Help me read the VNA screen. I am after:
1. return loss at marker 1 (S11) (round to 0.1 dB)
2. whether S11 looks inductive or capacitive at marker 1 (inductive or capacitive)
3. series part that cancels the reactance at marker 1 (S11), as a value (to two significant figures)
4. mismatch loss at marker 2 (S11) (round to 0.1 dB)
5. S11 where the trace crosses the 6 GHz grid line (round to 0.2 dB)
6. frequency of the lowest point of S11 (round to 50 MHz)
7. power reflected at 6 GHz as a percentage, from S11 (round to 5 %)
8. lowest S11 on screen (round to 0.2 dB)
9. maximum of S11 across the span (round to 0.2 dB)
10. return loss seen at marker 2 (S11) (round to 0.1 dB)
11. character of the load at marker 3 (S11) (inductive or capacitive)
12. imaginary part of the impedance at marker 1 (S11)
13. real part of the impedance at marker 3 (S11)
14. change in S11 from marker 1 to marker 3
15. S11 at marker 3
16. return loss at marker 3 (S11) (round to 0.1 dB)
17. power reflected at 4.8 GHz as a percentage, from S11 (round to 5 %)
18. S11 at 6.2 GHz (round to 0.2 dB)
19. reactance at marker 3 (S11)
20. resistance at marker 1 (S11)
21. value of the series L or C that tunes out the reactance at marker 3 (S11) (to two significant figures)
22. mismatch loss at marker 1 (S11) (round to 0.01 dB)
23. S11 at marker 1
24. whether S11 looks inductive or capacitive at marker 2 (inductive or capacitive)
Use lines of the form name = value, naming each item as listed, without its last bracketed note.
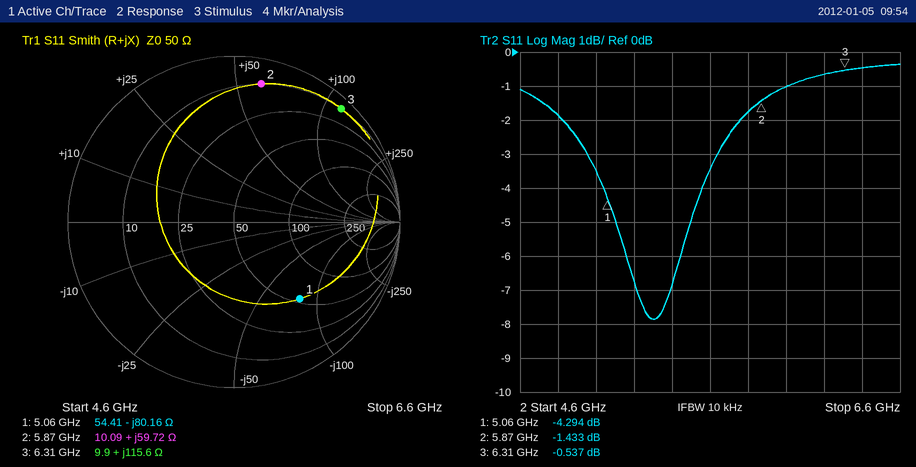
return loss at marker 1 (S11) = 4.3 dB
whether S11 looks inductive or capacitive at marker 1 = capacitive
series part that cancels the reactance at marker 1 (S11), as a value = 2.5 nH
mismatch loss at marker 2 (S11) = 5.5 dB
S11 where the trace crosses the 6 GHz grid line = -1.0 dB
frequency of the lowest point of S11 = 5.30 GHz
power reflected at 6 GHz as a percentage, from S11 = 80 %
lowest S11 on screen = -7.8 dB
maximum of S11 across the span = -0.4 dB
return loss seen at marker 2 (S11) = 1.4 dB
character of the load at marker 3 (S11) = inductive
imaginary part of the impedance at marker 1 = -80.16 Ω
real part of the impedance at marker 3 = 9.9 Ω
change in S11 from marker 1 to marker 3 = 3.757 dB
S11 at marker 3 = -0.537 dB
return loss at marker 3 (S11) = 0.5 dB
power reflected at 4.8 GHz as a percentage, from S11 = 65 %
S11 at 6.2 GHz = -0.6 dB
reactance at marker 3 = +115.6 Ω
resistance at marker 1 = 54.41 Ω
value of the series L or C that tunes out the reactance at marker 3 (S11) = 220 fF
mismatch loss at marker 1 (S11) = 2.02 dB
S11 at marker 1 = -4.294 dB
whether S11 looks inductive or capacitive at marker 2 = inductive
